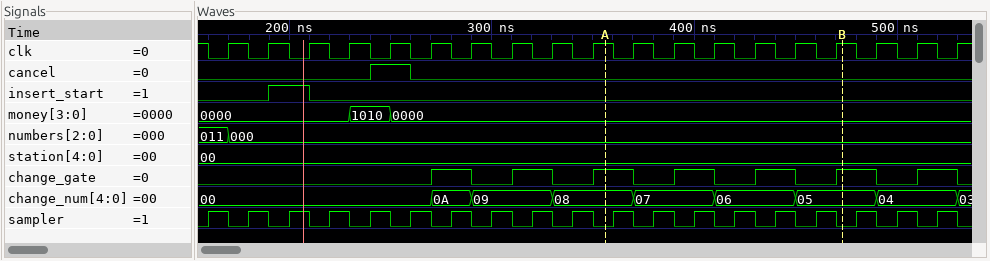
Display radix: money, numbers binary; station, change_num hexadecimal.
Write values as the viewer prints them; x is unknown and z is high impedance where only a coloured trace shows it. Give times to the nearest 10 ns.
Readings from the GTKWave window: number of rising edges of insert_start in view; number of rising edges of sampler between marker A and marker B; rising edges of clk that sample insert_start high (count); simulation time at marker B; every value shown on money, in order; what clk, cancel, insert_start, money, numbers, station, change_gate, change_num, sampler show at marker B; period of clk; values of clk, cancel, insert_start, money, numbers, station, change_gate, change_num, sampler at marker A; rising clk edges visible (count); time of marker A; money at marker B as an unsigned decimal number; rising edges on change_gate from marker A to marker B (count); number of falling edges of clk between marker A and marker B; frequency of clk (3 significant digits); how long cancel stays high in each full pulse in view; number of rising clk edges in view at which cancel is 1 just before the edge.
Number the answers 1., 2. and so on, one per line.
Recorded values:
1. 1
2. 6
3. 1
4. 470 ns
5. 0000, 1010, 0000
6. clk=1, cancel=0, insert_start=0, money=0000, numbers=000, station=00, change_gate=1, change_num=05, sampler=0
7. 20 ns
8. clk=1, cancel=0, insert_start=0, money=0000, numbers=000, station=00, change_gate=1, change_num=08, sampler=0
9. 19
10. 360 ns
11. 0
12. 3
13. 6
14. 50.0 MHz
15. 20 ns
16. 1
